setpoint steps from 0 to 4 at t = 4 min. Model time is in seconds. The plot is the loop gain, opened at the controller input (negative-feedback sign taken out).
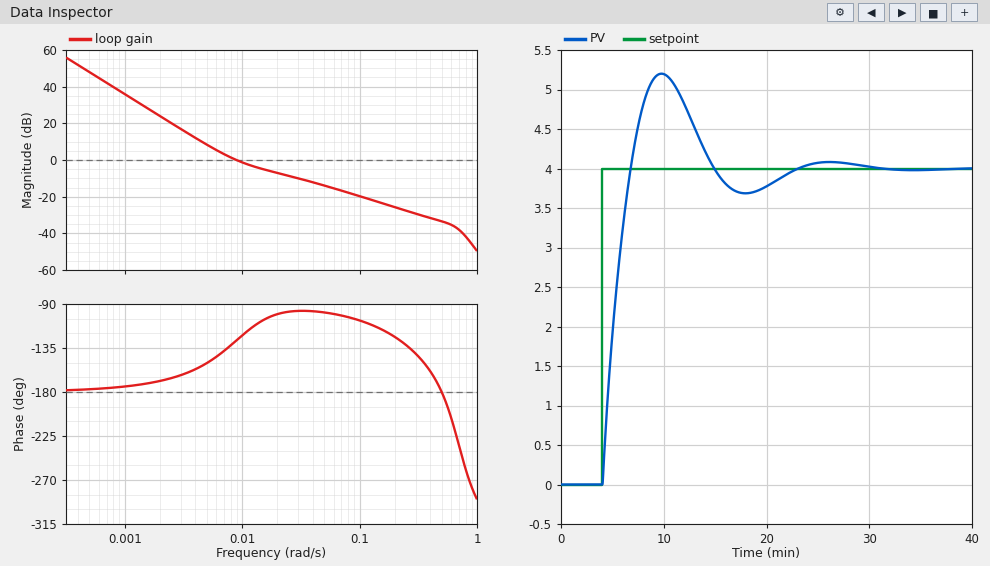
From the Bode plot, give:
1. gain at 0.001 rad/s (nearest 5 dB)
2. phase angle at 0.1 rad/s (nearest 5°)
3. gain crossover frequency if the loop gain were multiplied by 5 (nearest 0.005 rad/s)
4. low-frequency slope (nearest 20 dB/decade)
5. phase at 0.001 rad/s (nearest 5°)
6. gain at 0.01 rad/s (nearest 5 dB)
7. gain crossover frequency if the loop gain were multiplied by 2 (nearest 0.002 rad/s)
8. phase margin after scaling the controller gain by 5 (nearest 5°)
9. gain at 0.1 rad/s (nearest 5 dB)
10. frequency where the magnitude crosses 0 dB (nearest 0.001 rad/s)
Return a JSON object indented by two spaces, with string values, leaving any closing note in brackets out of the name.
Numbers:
{
  "gain at 0.001 rad/s": "35 dB",
  "phase angle at 0.1 rad/s": "-105°",
  "gain crossover frequency if the loop gain were multiplied by 5": "0.050 rad/s",
  "low-frequency slope": "-40 dB/decade",
  "phase at 0.001 rad/s": "-175°",
  "gain at 0.01 rad/s": "0 dB",
  "gain crossover frequency if the loop gain were multiplied by 2": "0.018 rad/s",
  "phase margin after scaling the controller gain by 5": "80°",
  "gain at 0.1 rad/s": "-20 dB",
  "frequency where the magnitude crosses 0 dB": "0.009 rad/s"
}
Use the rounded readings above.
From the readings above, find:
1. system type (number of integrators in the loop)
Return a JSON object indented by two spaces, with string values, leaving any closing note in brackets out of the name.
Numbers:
{
  "system type": "2"
}
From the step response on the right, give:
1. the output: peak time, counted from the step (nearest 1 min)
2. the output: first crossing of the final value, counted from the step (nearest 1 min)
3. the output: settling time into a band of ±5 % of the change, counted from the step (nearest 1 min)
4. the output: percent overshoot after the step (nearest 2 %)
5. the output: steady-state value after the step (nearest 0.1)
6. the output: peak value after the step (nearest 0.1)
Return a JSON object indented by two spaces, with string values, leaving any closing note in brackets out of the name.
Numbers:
{
  "the output: peak time, counted from the step": "6 min",
  "the output: first crossing of the final value, counted from the step": "3 min",
  "the output: settling time into a band of ±5 % of the change, counted from the step": "16 min",
  "the output: percent overshoot after the step": "30 %",
  "the output: steady-state value after the step": "4.0",
  "the output: peak value after the step": "5.2"
}
